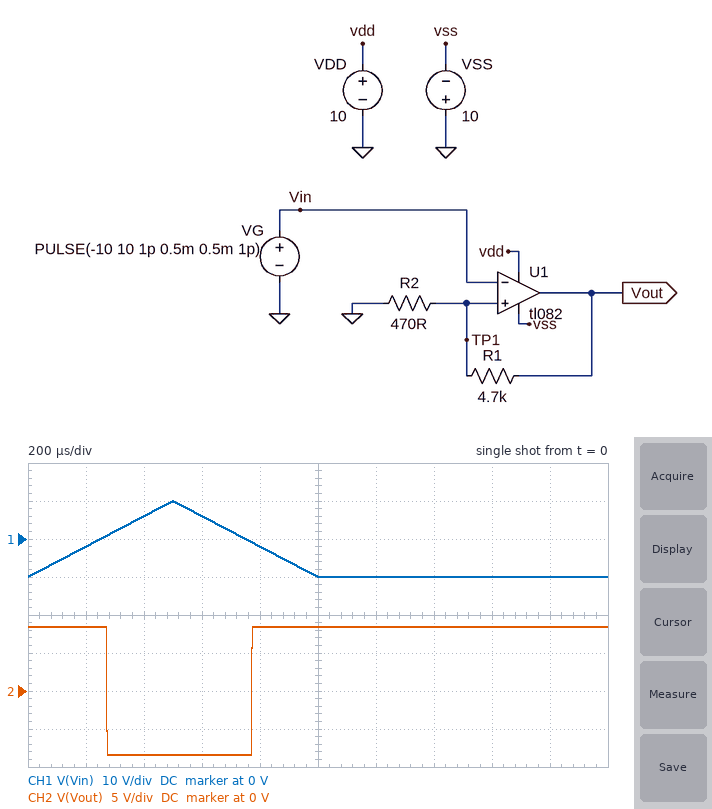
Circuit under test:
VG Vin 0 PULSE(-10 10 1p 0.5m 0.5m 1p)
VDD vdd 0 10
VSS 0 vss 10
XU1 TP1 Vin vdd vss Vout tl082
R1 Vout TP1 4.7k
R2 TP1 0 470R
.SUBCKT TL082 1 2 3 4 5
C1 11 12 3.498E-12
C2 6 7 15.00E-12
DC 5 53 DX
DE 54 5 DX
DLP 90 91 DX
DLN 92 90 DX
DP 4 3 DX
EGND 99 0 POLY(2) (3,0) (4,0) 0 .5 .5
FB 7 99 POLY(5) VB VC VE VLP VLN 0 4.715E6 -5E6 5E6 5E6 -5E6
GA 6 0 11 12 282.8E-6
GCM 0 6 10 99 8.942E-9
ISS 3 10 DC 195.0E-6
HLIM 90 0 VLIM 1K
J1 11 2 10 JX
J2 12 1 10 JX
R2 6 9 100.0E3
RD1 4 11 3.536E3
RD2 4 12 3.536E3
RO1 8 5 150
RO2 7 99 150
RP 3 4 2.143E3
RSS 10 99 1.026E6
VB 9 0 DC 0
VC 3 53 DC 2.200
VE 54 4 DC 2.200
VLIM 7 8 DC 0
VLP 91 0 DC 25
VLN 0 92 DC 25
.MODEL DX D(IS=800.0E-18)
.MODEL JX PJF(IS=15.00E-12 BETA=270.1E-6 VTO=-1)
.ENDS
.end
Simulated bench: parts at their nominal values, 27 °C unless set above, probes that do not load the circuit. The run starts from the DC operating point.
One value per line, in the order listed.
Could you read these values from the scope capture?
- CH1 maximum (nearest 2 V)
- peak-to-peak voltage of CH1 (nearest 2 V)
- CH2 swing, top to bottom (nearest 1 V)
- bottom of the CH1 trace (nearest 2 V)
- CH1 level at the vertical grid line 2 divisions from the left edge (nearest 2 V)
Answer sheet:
10 V
20 V
17 V
-10 V
6 V
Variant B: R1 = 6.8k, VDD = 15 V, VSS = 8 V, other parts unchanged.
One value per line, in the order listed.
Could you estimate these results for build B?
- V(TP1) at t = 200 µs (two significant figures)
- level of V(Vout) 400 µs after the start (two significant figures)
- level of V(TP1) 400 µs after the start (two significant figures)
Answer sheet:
870 mV
-6.5 V
-420 mV
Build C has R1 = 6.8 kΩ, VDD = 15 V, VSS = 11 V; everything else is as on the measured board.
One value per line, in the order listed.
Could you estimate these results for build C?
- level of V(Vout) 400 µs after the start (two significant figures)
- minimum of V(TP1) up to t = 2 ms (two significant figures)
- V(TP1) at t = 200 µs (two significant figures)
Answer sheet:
-9.5 V
-610 mV
870 mV
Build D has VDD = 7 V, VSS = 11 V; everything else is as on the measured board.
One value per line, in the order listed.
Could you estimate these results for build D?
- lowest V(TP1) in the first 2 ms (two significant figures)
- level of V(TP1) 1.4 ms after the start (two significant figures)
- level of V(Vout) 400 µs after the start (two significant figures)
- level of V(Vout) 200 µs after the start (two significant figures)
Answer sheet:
-860 mV
500 mV
-9.5 V
5.5 V
